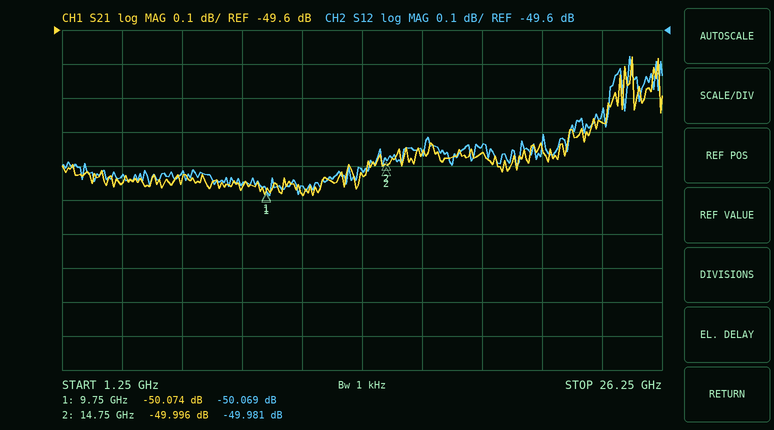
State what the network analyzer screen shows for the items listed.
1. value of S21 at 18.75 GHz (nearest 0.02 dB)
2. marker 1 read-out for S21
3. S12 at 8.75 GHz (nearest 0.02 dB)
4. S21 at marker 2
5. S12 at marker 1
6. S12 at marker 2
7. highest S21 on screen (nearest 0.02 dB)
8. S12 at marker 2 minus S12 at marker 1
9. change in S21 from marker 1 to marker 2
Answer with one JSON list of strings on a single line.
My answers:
["-49.96 dB", "-50.074 dB", "-50.06 dB", "-49.996 dB", "-50.069 dB", "-49.981 dB", "-49.68 dB", "0.088 dB", "0.078 dB"]
